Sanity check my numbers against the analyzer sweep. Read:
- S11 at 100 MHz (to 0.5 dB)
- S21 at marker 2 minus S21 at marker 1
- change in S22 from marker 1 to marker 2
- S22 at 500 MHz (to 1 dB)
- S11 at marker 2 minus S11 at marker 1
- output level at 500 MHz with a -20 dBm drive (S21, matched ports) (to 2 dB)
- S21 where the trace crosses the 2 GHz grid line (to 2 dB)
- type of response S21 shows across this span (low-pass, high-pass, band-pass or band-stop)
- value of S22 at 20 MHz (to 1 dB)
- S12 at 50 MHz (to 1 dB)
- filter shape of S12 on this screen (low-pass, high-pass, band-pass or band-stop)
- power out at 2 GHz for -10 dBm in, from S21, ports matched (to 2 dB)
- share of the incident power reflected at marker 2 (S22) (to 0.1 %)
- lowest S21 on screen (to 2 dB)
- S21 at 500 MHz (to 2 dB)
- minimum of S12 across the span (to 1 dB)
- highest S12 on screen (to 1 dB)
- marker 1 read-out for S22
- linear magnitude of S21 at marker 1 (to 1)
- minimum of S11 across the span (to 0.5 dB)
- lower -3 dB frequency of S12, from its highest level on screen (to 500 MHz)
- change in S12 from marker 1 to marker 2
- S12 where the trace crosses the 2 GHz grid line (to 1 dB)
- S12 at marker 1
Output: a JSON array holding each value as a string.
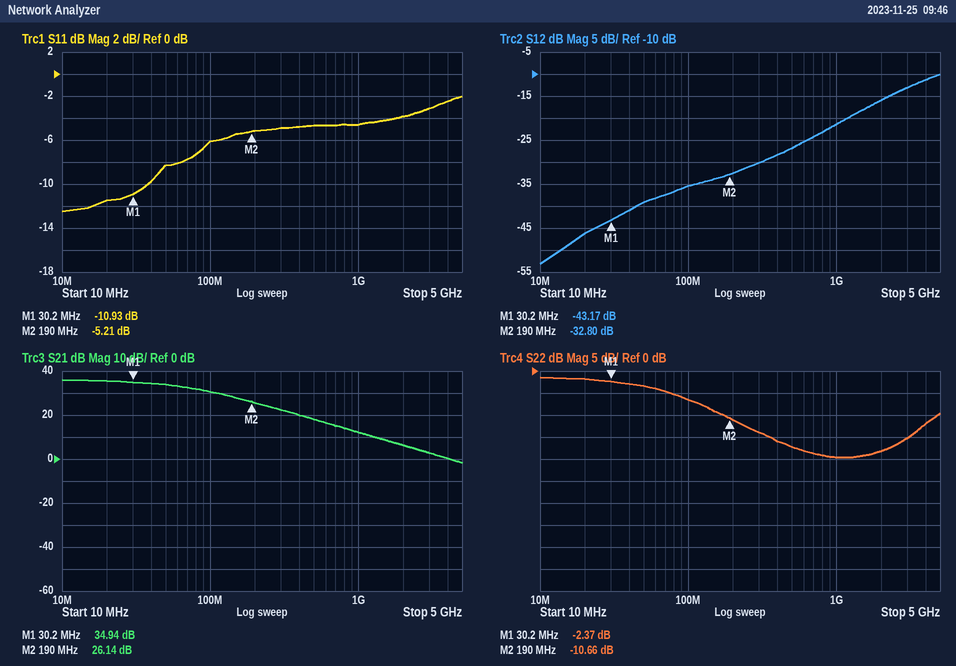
["-6.0 dB", "-8.80 dB", "-8.29 dB", "-17 dB", "5.72 dB", "-2 dBm", "6 dB", "low-pass", "-2 dB", "-39 dB", "high-pass", "-4 dBm", "8.6 %", "-2 dB", "18 dB", "-53 dB", "-10 dB", "-2.37 dB", "56", "-12.5 dB", "3.0 GHz", "10.37 dB", "-16 dB", "-43.17 dB"]
